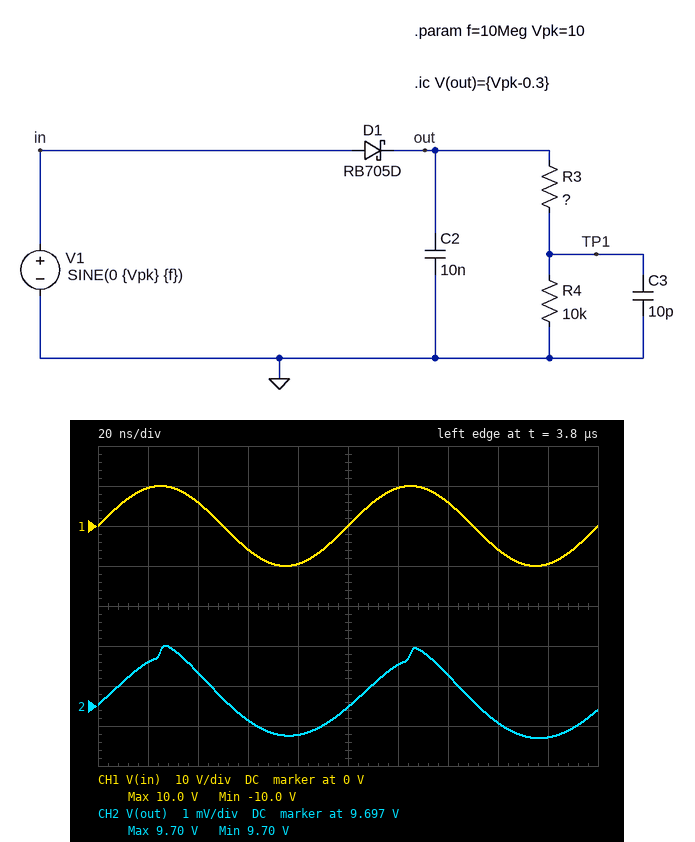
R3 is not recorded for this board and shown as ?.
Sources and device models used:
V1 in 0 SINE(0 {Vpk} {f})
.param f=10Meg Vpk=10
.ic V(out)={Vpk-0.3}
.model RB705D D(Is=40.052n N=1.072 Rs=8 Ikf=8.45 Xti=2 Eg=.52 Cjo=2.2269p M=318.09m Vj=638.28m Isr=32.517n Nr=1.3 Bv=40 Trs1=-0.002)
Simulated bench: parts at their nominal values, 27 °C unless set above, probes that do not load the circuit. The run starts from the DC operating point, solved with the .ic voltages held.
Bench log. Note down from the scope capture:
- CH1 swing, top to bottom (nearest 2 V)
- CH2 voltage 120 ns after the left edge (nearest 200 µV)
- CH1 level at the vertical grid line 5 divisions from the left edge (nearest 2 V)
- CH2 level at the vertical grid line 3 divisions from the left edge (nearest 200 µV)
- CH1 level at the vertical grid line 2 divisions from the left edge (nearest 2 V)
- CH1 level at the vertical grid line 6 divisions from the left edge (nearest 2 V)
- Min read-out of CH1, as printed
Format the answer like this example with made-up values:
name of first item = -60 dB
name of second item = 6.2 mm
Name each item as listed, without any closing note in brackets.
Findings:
CH1 swing, top to bottom = 20 V
CH2 voltage 120 ns after the left edge = 9.6980 V
CH1 level at the vertical grid line 5 divisions from the left edge = 0 V
CH2 level at the vertical grid line 3 divisions from the left edge = 9.6966 V
CH1 level at the vertical grid line 2 divisions from the left edge = 6 V
CH1 level at the vertical grid line 6 divisions from the left edge = 10 V
Min read-out of CH1, as printed = -10.0 V
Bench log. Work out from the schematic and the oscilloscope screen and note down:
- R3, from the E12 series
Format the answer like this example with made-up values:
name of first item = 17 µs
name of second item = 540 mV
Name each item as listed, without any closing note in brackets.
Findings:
R3, from the E12 series = 220 kΩ
